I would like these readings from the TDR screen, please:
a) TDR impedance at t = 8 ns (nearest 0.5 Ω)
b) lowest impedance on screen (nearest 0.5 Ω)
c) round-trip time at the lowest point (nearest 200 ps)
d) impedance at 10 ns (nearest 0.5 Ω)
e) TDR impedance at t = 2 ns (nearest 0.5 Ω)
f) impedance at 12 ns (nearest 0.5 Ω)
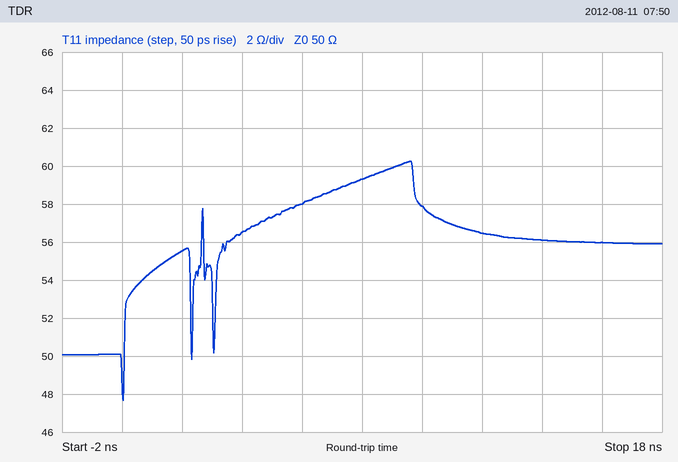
59.5 Ω
47.5 Ω
0.0 ns
58.0 Ω
55.5 Ω
56.5 Ω
